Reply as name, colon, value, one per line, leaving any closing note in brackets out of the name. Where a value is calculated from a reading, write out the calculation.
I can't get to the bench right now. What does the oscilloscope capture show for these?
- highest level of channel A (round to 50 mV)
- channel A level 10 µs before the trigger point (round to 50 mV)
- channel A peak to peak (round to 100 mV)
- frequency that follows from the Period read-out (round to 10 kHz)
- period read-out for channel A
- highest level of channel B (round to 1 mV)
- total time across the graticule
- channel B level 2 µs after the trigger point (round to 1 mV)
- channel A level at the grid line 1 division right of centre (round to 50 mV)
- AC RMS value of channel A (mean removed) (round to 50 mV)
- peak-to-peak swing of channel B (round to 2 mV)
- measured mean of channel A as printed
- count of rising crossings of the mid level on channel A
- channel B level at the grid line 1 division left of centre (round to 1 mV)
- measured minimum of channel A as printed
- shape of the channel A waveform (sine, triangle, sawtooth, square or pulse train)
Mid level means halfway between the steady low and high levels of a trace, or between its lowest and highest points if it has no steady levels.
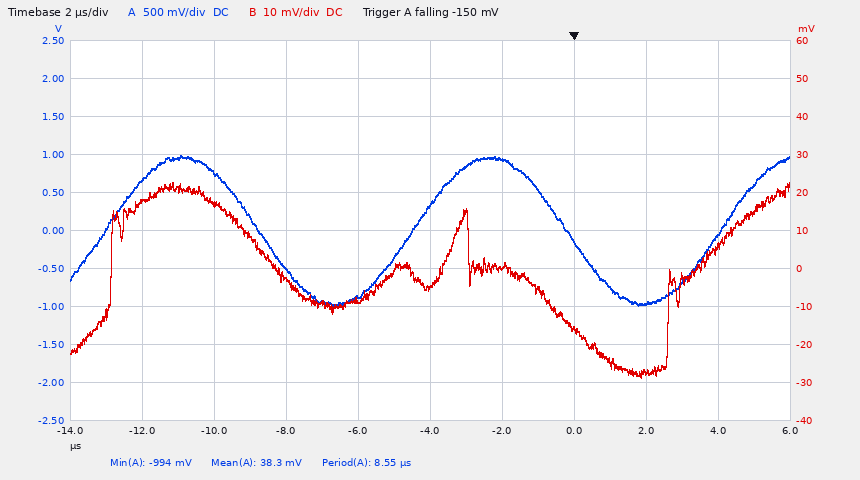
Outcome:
highest level of channel A: 1.00 V
channel A level 10 µs before the trigger point: 750 mV
channel A peak to peak: 2.00 V
frequency that follows from the Period read-out: 1 / 8.55 µs ≈ 117 kHz, so 120 kHz to the nearest 10 kHz
period read-out for channel A: 8.55 µs
highest level of channel B: 23 mV
total time across the graticule: 20 µs
channel B level 2 µs after the trigger point: -27 mV
channel A level at the grid line 1 division right of centre: 950 mV
AC RMS value of channel A (mean removed): 2.00 V / (2√2) ≈ 707 mV, so 700 mV to the nearest 50 mV
peak-to-peak swing of channel B: 52 mV
measured mean of channel A as printed: 38.3 mV
count of rising crossings of the mid level on channel A: 3
channel B level at the grid line 1 division left of centre: -8 mV
measured minimum of channel A as printed: -994 mV
shape of the channel A waveform: sine
